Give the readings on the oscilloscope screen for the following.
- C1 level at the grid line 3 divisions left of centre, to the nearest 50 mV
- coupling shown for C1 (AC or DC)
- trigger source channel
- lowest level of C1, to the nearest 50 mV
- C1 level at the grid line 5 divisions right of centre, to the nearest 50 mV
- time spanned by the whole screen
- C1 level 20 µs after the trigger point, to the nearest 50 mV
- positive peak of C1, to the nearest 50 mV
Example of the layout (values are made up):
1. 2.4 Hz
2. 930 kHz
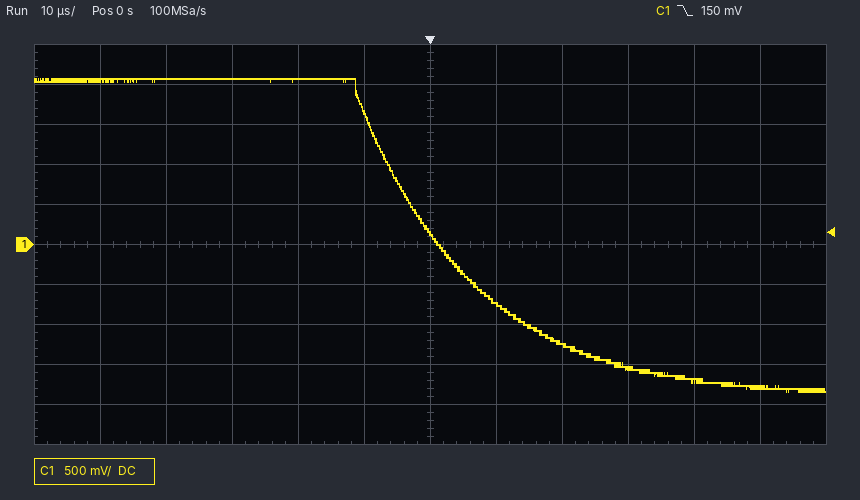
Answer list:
1. 2.10 V
2. DC
3. C1
4. -1.85 V
5. -1.80 V
6. 120 µs
7. -1.25 V
8. 2.10 V
